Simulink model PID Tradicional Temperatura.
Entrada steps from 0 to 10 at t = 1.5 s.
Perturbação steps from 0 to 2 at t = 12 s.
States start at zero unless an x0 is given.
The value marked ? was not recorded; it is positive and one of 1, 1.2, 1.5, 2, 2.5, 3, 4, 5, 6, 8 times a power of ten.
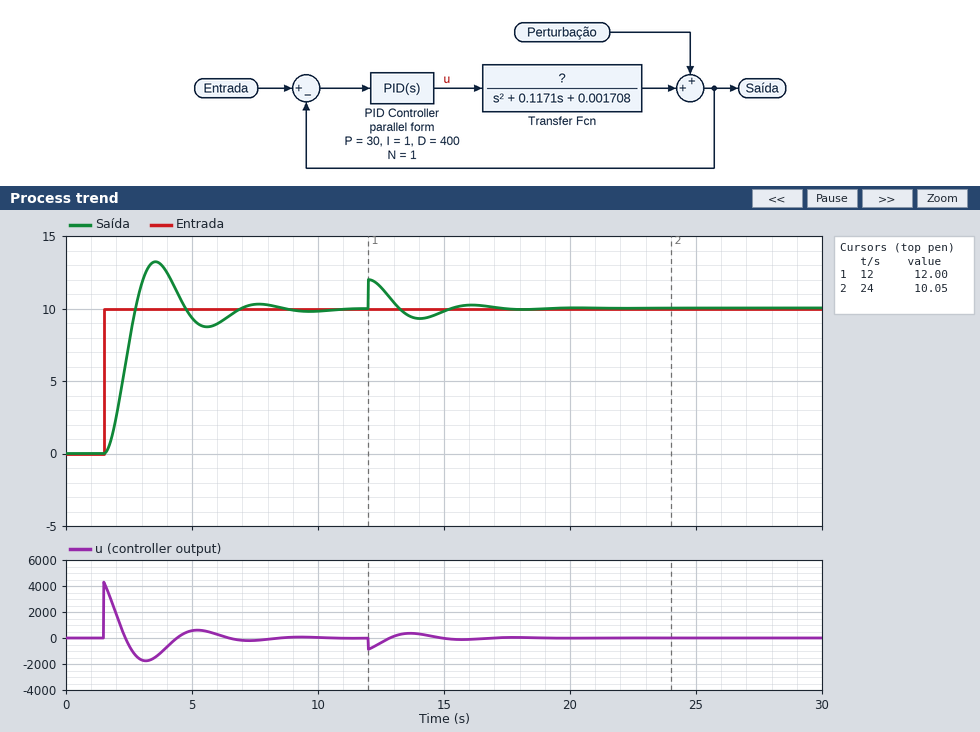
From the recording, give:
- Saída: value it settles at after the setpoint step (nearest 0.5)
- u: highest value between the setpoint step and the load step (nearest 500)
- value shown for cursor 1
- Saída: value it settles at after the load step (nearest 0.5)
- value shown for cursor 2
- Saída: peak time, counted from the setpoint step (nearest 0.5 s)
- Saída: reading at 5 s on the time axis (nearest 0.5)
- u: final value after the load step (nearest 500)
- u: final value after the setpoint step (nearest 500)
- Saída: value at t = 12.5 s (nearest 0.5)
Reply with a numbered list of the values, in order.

1. 10.0
2. 4500
3. 12.00
4. 10.0
5. 10.05
6. 2.0 s
7. 9.5
8. 0
9. 0
10. 11.5
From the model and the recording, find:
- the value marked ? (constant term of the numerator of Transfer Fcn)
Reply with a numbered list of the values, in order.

1. 0.006
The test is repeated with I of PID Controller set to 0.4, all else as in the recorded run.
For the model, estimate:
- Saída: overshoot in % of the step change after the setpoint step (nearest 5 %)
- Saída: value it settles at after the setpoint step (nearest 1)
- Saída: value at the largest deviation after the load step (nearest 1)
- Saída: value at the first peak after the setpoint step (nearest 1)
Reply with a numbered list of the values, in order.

1. 30 %
2. 10
3. 12
4. 13
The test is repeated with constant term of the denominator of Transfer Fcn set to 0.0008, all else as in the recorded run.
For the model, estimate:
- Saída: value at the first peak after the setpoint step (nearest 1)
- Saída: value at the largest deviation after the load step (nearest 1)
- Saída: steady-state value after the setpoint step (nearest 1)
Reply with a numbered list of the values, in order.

1. 13
2. 12
3. 10
